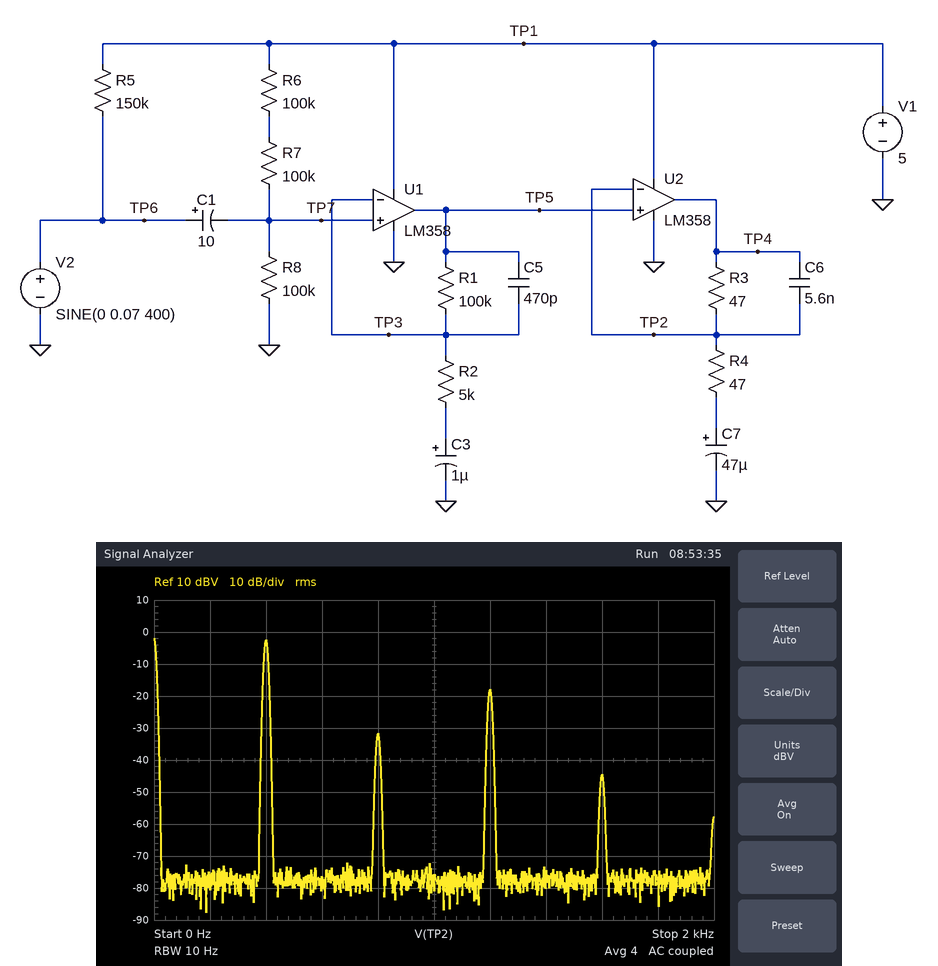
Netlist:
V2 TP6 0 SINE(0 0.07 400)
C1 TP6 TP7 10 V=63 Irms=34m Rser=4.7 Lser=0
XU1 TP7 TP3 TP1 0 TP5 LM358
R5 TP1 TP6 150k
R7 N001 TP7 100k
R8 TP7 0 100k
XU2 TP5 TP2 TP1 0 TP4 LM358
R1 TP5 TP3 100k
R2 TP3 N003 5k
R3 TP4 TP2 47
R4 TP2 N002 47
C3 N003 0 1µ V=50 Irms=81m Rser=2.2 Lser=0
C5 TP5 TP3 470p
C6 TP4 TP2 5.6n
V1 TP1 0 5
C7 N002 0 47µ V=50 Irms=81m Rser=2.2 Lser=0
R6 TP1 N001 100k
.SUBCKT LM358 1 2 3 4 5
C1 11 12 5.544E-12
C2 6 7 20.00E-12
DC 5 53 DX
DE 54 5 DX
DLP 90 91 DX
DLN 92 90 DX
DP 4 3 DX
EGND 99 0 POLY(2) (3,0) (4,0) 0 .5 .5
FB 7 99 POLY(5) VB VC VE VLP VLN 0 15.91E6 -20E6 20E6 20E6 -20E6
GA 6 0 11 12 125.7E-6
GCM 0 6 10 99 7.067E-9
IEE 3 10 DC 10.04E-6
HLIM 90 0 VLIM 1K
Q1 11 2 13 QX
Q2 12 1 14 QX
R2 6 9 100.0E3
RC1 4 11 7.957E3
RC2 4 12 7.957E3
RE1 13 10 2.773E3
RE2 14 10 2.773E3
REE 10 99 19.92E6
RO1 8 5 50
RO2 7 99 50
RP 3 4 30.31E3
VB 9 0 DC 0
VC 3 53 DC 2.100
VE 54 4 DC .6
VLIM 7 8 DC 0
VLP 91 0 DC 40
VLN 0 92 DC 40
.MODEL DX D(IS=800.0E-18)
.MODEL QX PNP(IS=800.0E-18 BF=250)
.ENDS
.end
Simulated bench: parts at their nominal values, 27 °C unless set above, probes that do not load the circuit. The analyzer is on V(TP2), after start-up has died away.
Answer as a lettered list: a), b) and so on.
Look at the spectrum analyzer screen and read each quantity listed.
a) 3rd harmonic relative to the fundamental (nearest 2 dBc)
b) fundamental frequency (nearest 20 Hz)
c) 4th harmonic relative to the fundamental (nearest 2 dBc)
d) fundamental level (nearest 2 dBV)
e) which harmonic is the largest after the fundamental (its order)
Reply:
a) -16 dBc
b) 400 Hz
c) -42 dBc
d) -2 dBV
e) 3
